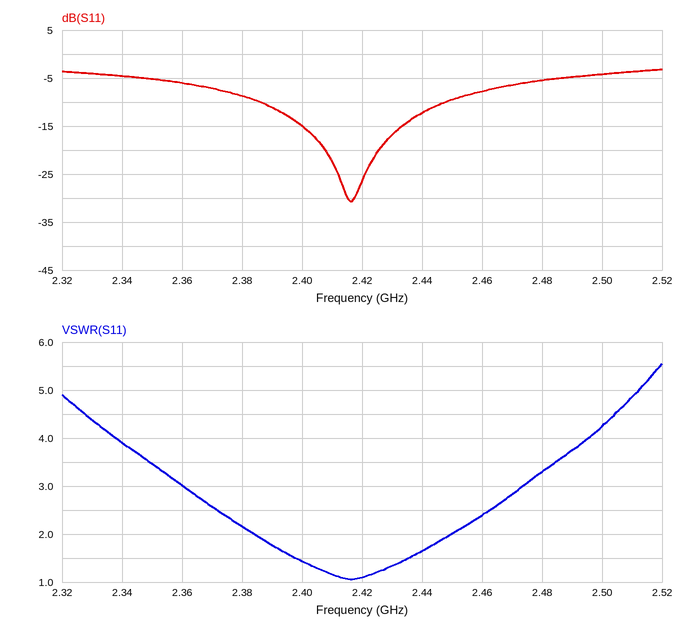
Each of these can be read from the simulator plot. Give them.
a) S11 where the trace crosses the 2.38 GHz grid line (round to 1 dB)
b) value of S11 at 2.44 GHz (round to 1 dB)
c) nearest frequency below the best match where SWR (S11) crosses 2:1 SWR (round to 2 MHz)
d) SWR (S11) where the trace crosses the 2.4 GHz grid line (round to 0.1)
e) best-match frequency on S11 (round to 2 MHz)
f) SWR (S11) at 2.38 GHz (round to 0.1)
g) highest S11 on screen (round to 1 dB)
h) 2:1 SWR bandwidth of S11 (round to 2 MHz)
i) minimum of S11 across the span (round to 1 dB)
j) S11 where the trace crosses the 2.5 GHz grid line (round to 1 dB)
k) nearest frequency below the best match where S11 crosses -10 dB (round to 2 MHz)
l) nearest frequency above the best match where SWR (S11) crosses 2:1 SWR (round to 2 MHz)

-9 dB
-12 dB
2.384 GHz
1.4
2.416 GHz
2.2
-3 dB
66 MHz
-31 dB
-4 dB
2.386 GHz
2.450 GHz
